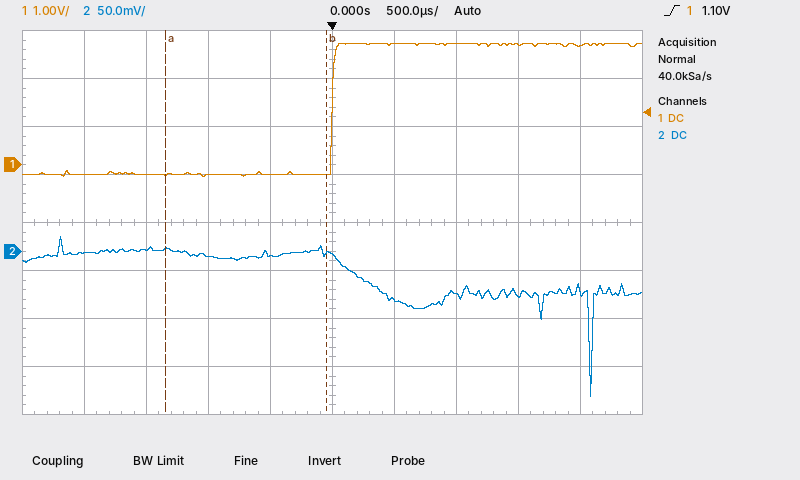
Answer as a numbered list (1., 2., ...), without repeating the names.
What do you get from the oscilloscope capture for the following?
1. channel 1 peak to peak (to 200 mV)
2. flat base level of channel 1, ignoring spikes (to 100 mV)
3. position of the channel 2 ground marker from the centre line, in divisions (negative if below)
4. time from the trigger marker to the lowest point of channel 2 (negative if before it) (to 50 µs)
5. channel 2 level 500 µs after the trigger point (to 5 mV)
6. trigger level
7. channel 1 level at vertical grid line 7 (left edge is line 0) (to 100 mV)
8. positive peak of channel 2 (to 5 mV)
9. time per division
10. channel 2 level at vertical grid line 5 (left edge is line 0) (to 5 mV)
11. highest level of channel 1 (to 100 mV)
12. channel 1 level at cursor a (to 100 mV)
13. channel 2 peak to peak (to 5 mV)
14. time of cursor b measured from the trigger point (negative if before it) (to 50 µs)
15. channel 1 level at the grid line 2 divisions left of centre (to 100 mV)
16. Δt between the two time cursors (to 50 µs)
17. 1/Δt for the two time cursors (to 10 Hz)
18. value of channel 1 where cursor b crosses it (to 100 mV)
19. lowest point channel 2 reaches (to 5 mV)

1. 2.8 V
2. -200 mV
3. -0.6 div
4. +2.10 ms
5. -50 mV
6. 1.10 V
7. 2.5 V
8. 15 mV
9. 500 µs
10. -5 mV
11. 2.5 V
12. -200 mV
13. 165 mV
14. -50 µs
15. -200 mV
16. 1.30 ms
17. 770 Hz
18. -200 mV
19. -150 mV
